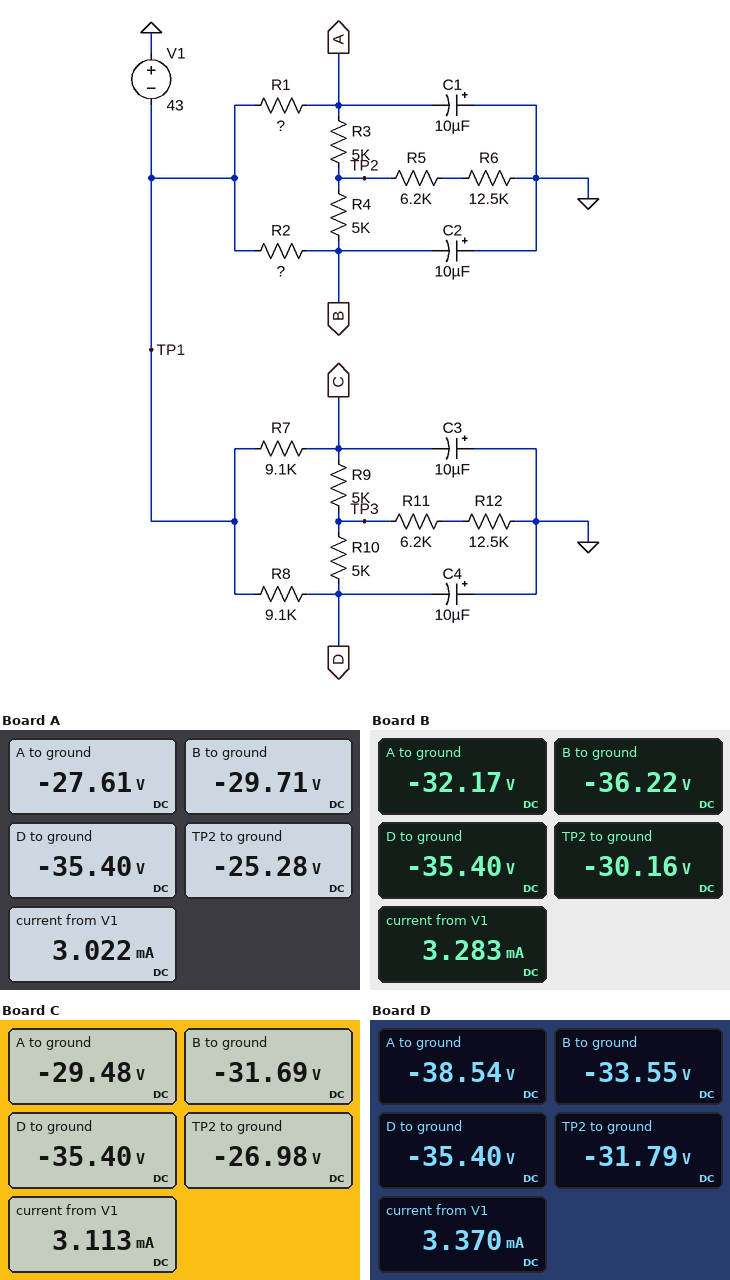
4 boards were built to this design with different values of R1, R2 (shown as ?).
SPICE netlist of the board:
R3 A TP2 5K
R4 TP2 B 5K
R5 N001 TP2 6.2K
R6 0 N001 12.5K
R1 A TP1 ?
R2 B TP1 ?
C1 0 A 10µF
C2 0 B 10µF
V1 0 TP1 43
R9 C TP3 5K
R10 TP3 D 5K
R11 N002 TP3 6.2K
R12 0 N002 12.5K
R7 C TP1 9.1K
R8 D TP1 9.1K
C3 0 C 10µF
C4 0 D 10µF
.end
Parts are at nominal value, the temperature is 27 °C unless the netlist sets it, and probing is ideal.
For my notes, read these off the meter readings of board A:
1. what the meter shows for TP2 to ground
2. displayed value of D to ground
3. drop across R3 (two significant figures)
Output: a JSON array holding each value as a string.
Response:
["-25.28 V", "-35.40 V", "2.3 V"]
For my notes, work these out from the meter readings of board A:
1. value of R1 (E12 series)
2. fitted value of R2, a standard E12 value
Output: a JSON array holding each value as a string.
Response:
["33 kΩ", "15 kΩ"]
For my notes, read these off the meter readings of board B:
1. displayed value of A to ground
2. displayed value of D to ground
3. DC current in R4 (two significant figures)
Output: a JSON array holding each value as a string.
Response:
["-32.17 V", "-35.40 V", "1.2 mA"]
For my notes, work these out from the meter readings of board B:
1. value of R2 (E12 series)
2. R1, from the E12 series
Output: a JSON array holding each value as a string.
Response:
["5.6 kΩ", "27 kΩ"]
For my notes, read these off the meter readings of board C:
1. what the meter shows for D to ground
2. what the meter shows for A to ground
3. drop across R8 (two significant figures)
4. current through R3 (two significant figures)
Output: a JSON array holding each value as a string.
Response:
["-35.40 V", "-29.48 V", "7.6 V", "500 µA"]
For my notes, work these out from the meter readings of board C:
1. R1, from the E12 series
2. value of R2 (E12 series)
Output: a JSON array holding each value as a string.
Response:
["27 kΩ", "12 kΩ"]
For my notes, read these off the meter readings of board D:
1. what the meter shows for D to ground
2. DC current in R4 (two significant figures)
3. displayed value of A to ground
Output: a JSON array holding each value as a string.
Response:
["-35.40 V", "350 µA", "-38.54 V"]
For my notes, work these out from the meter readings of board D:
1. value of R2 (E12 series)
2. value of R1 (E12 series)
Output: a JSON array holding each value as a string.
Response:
["27 kΩ", "3.3 kΩ"]
